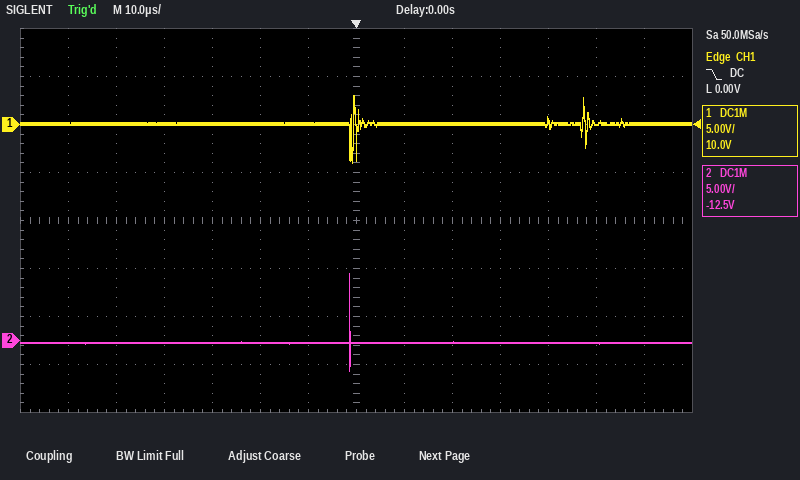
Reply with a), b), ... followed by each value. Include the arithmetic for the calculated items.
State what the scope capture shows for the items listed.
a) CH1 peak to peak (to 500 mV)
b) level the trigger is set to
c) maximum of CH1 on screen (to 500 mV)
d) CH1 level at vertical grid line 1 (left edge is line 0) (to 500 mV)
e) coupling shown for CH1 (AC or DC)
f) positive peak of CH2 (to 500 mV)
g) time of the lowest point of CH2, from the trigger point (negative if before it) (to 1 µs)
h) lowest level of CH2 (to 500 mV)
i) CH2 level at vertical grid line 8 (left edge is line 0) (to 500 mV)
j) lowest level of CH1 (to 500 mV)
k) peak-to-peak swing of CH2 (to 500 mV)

a) 3.0 V − (-4.0 V) = 7.0 V
b) 0.00 V
c) 3.0 V
d) 0.0 V
e) DC
f) 7.0 V
g) -1 µs
h) -3.0 V
i) 0.0 V
j) -4.0 V
k) 7.0 V − (-3.0 V) = 10.0 V
